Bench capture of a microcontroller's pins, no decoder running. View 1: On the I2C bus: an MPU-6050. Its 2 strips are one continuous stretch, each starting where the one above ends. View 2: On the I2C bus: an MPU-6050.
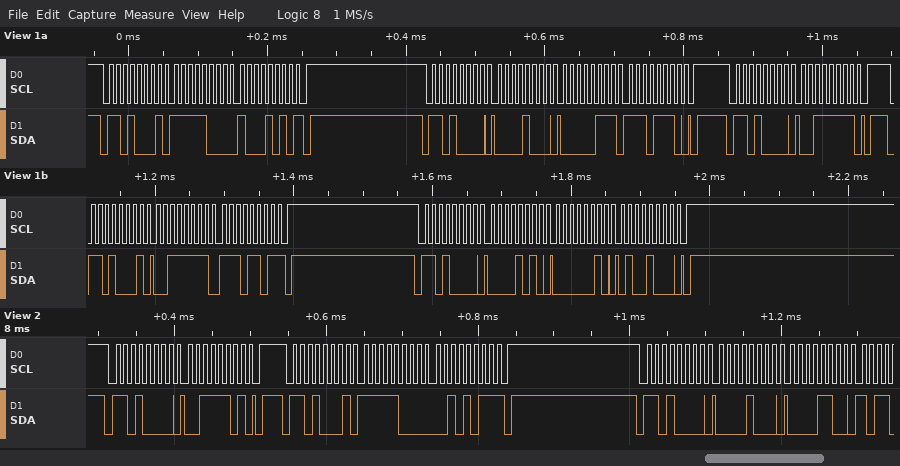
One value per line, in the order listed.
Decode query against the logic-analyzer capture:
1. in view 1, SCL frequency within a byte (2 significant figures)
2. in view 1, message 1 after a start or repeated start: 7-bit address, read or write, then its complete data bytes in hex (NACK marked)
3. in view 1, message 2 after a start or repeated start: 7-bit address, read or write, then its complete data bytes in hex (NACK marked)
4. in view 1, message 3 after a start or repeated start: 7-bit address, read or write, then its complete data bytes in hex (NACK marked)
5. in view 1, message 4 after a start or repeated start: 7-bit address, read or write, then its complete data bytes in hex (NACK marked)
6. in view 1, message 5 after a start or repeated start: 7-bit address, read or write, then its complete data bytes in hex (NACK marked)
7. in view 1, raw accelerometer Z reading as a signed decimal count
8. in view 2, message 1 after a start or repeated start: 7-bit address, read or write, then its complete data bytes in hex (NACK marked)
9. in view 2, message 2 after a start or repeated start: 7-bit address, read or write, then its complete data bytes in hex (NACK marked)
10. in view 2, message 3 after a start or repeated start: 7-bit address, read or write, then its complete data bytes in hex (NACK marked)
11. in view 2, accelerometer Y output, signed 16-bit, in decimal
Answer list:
100 kHz
0x68 read: F8 8A NACK
0x68 write: 08 07 EE
0x68 write: 3F
0x68 read: 3F ED NACK
0x68 write: 0A 02 48
16365
0x68 write: 3D
0x68 read: F8 2B NACK
0x68 write: 08 0C
-2005
